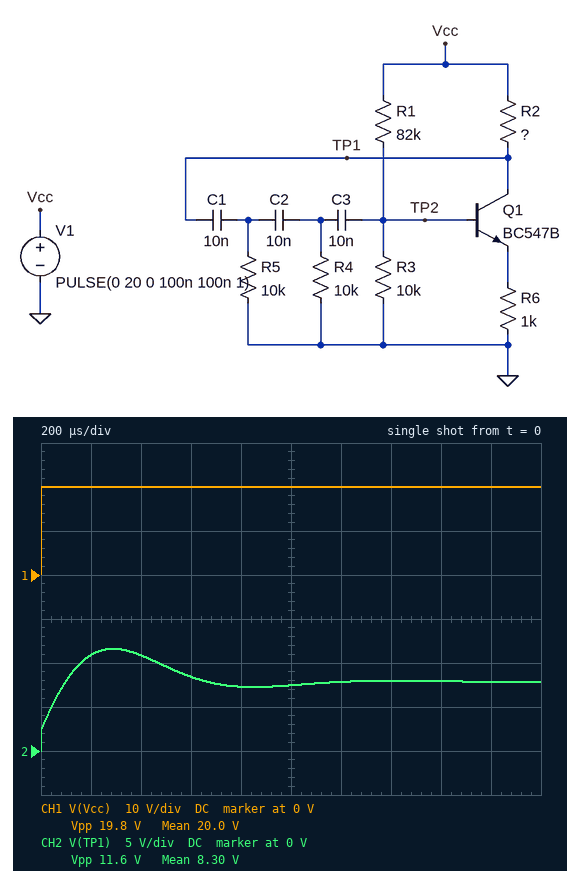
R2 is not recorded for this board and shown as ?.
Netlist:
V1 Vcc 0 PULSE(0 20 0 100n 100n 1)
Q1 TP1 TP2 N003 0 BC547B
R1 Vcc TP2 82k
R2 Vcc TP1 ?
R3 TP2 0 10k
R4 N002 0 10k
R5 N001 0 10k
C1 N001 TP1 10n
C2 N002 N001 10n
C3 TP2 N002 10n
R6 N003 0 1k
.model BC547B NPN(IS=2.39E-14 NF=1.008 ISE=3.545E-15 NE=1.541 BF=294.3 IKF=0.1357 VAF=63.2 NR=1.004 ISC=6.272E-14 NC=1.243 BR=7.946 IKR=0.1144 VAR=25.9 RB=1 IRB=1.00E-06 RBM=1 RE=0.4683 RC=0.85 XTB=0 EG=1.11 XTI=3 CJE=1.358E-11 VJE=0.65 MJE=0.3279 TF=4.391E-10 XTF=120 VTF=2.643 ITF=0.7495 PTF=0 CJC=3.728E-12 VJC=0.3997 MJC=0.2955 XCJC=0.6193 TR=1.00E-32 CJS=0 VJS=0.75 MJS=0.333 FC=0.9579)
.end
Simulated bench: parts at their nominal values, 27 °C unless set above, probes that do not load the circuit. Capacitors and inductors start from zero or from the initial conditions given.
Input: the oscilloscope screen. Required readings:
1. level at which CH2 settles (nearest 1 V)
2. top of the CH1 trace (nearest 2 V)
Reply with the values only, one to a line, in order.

8 V
20 V
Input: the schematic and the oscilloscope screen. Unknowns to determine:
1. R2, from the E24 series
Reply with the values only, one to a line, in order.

8.2 kΩ
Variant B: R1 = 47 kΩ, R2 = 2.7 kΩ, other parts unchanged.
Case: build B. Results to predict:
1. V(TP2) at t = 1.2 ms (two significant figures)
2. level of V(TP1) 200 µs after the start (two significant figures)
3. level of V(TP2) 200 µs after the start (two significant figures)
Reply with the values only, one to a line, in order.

3.4 V
15 V
2.2 V
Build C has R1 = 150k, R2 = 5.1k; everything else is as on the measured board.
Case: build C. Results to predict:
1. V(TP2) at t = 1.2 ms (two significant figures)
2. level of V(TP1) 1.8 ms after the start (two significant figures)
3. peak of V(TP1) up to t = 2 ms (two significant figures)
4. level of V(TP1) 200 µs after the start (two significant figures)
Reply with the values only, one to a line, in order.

1.2 V
17 V
19 V
18 V
